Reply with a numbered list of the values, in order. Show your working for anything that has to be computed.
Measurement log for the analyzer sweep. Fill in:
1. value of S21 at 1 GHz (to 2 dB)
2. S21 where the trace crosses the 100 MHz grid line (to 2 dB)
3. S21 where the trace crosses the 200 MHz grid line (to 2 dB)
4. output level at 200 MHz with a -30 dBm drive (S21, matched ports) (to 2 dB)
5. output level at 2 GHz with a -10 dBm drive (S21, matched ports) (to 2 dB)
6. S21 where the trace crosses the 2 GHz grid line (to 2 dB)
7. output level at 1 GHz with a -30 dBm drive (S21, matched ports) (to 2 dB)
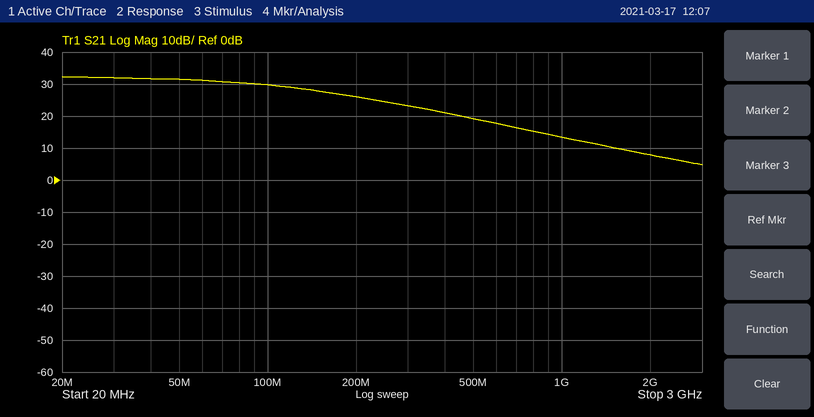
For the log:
1. 14 dB
2. 30 dB
3. 26 dB
4. -30 dBm + (26 dB) = -4 dBm
5. -10 dBm + (8 dB) = -2 dBm
6. 8 dB
7. -30 dBm + (14 dB) = -16 dBm
